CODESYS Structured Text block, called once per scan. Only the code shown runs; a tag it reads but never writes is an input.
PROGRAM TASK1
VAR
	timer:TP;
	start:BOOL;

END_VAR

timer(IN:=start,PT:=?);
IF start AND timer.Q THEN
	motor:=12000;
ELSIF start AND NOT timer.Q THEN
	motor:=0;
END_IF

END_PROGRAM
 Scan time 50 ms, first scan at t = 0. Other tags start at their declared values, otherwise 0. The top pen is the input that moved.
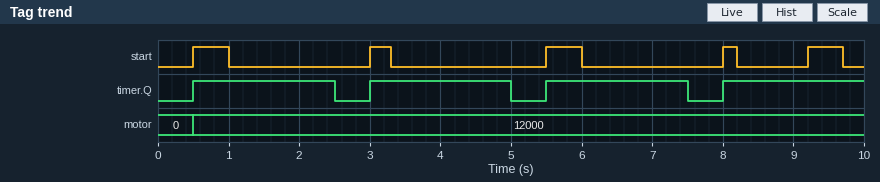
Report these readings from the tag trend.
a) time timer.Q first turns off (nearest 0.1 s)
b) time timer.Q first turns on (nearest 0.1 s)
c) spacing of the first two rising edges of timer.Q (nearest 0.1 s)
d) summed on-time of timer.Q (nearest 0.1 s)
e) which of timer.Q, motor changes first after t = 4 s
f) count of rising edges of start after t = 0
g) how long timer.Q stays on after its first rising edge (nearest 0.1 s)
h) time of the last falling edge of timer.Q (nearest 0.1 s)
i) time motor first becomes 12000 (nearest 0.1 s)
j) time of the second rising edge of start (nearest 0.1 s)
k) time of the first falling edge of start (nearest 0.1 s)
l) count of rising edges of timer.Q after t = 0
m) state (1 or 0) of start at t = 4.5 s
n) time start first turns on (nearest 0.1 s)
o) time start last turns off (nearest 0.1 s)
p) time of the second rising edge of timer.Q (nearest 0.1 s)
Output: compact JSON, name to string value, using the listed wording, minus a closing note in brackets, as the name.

{"time timer.Q first turns off": "2.5 s", "time timer.Q first turns on": "0.5 s", "spacing of the first two rising edges of timer.Q": "2.5 s", "summed on-time of timer.Q": "8.0 s", "which of timer.Q, motor changes first after t = 4 s": "timer.Q", "count of rising edges of start after t = 0": "5", "how long timer.Q stays on after its first rising edge": "2.0 s", "time of the last falling edge of timer.Q": "7.5 s", "time motor first becomes 12000": "0.5 s", "time of the second rising edge of start": "3.0 s", "time of the first falling edge of start": "1.0 s", "count of rising edges of timer.Q after t = 0": "4", "state (1 or 0) of start at t = 4.5 s": "0", "time start first turns on": "0.5 s", "time start last turns off": "9.7 s", "time of the second rising edge of timer.Q": "3.0 s"}
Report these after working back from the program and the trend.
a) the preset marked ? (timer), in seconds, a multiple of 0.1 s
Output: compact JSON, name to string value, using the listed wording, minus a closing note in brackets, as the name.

{"the preset marked ? (timer), in seconds, a multiple of 0.1 s": "2.0 s"}
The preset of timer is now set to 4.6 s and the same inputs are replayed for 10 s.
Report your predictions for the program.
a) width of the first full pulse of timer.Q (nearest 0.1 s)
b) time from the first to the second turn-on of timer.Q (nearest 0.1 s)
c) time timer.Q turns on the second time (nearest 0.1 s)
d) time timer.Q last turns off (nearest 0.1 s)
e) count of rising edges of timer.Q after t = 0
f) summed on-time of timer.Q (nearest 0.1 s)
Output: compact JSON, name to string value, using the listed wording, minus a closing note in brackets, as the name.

{"width of the first full pulse of timer.Q": "4.6 s", "time from the first to the second turn-on of timer.Q": "5.0 s", "time timer.Q turns on the second time": "5.5 s", "time timer.Q last turns off": "5.1 s", "count of rising edges of timer.Q after t = 0": "2", "summed on-time of timer.Q": "9.1 s"}
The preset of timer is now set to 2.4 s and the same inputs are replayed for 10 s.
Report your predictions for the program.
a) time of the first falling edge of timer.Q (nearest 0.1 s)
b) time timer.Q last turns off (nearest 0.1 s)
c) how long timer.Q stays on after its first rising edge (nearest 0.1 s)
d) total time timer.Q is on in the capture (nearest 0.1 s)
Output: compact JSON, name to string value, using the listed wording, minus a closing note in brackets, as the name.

{"time of the first falling edge of timer.Q": "2.9 s", "time timer.Q last turns off": "7.9 s", "how long timer.Q stays on after its first rising edge": "2.4 s", "total time timer.Q is on in the capture": "9.2 s"}
